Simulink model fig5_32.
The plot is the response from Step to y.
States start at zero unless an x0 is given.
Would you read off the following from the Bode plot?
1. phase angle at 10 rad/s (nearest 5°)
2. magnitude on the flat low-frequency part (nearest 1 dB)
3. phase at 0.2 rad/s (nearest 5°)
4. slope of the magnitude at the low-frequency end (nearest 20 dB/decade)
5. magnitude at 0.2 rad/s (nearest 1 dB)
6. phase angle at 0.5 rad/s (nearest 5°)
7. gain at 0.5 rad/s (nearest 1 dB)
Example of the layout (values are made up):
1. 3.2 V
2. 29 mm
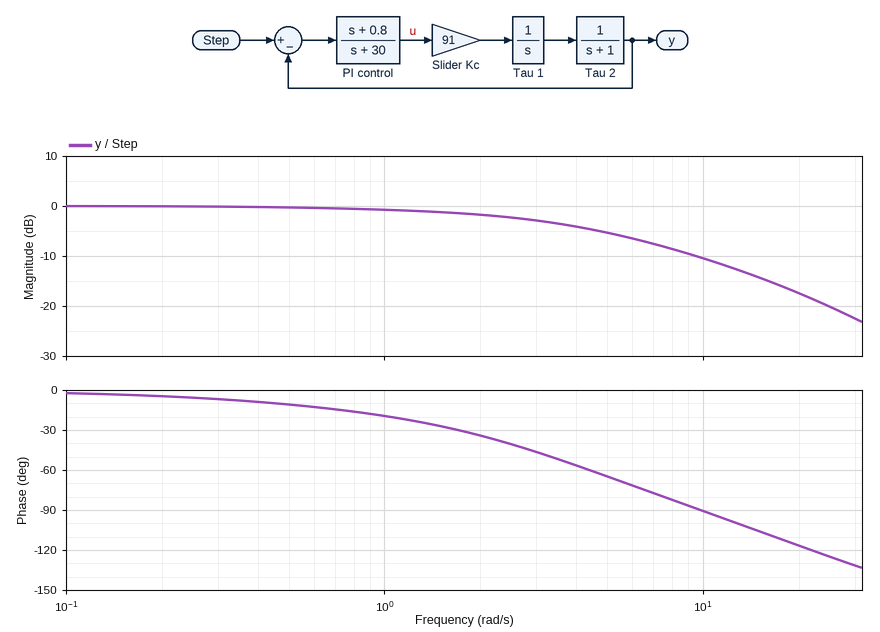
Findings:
1. -90°
2. 0 dB
3. -5°
4. 0 dB/decade
5. 0 dB
6. -10°
7. 0 dB
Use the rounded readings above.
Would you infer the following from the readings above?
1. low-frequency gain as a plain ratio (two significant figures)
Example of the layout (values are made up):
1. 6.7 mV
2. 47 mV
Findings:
1. 1.0
